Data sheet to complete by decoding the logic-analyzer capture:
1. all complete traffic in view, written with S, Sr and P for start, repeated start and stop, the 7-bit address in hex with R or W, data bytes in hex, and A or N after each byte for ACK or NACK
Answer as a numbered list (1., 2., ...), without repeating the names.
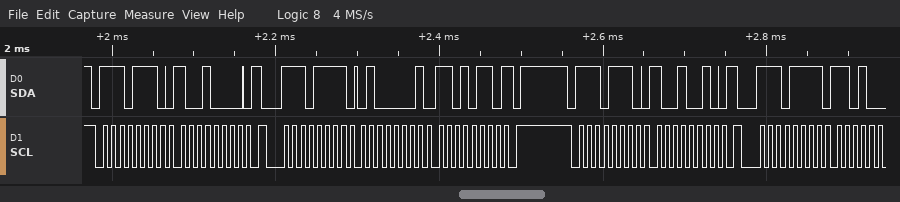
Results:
1. S 77W A 90 A Sr 77R A 41 A D6 N P S 77W A 92 A Sr 77R A
